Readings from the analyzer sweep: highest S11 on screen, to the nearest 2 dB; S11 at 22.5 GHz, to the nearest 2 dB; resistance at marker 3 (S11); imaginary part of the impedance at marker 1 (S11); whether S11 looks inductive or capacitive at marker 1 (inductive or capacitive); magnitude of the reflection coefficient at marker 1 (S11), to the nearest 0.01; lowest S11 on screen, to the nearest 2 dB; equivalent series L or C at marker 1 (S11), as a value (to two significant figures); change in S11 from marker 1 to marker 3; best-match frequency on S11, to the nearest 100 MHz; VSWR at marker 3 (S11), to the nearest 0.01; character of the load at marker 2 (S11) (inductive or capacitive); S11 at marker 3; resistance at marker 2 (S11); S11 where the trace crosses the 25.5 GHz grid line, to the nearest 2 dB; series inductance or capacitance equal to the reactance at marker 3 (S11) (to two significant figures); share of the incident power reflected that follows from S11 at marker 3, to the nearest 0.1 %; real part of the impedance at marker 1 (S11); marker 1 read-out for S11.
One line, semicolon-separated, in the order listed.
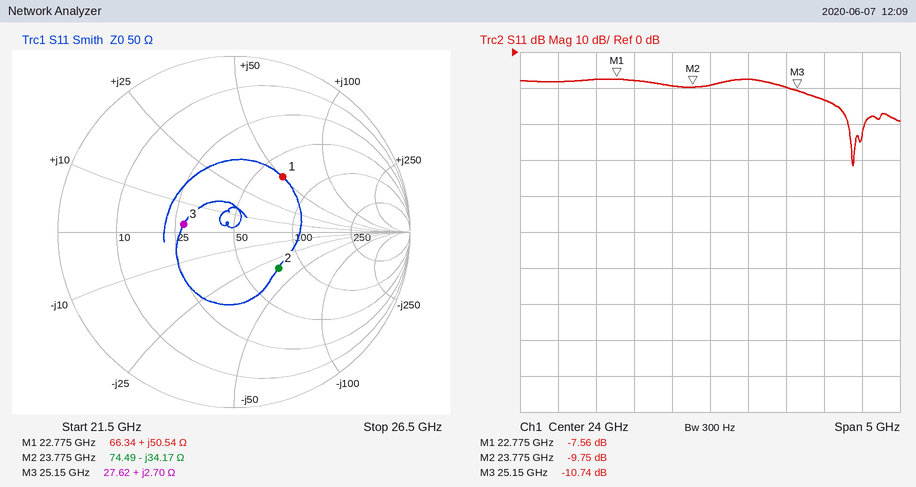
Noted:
-8 dB; -8 dB; 27.62 Ω; +50.54 Ω; inductive; 0.42; -32 dB; 350 pH; -3.18 dB; 25.9 GHz; 1.82; capacitive; -10.74 dB; 74.49 Ω; -14 dB; 17 pH; 8.4 %; 66.34 Ω; -7.56 dB
